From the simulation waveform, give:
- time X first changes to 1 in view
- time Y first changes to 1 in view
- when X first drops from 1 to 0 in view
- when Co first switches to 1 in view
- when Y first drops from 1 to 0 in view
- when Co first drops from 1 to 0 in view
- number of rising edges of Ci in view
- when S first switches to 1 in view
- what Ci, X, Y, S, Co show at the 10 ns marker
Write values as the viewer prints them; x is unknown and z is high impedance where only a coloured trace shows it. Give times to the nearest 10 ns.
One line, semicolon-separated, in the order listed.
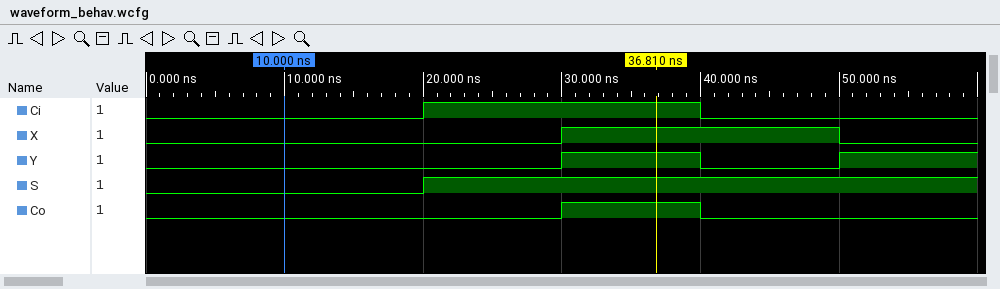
30 ns; 30 ns; 50 ns; 30 ns; 40 ns; 40 ns; 1; 20 ns; Ci=0, X=0, Y=0, S=0, Co=0
